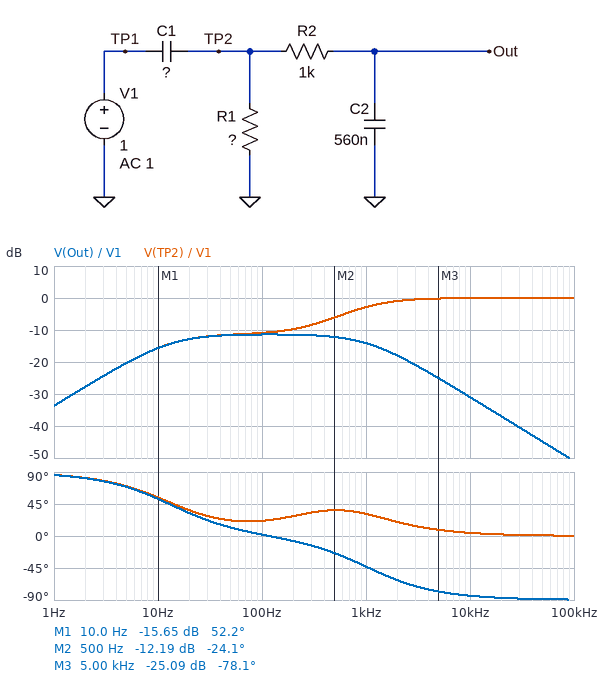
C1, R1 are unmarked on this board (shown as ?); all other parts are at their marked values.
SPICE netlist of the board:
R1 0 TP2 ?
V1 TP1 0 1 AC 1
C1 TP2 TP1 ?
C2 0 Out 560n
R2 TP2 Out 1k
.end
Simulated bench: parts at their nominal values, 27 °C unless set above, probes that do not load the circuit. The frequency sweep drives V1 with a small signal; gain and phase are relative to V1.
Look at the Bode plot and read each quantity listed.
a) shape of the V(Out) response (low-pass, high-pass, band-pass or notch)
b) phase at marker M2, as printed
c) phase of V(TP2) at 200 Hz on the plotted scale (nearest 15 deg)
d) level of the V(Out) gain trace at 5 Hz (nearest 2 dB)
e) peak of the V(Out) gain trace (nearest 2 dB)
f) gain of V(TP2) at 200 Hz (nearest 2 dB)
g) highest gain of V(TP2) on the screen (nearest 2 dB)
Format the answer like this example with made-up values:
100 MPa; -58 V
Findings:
band-pass; -24.1 deg; 30 deg; -20 dB; -12 dB; -10 dB; 0 dB
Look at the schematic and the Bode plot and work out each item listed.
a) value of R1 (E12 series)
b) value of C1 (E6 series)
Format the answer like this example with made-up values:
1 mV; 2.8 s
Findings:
15 kΩ; 220 nF
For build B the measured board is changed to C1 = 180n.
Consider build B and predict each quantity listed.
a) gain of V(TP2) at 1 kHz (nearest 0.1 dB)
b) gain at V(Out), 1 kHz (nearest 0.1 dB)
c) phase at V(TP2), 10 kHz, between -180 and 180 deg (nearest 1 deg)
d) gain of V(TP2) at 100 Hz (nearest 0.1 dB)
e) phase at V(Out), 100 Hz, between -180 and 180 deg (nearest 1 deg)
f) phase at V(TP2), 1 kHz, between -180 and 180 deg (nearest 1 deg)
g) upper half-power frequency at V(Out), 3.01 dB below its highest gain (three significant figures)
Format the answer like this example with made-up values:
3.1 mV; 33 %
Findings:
-3.6 dB; -14.9 dB; 5 deg; -12.2 dB; 3 deg; 35 deg; 1.24 kHz
